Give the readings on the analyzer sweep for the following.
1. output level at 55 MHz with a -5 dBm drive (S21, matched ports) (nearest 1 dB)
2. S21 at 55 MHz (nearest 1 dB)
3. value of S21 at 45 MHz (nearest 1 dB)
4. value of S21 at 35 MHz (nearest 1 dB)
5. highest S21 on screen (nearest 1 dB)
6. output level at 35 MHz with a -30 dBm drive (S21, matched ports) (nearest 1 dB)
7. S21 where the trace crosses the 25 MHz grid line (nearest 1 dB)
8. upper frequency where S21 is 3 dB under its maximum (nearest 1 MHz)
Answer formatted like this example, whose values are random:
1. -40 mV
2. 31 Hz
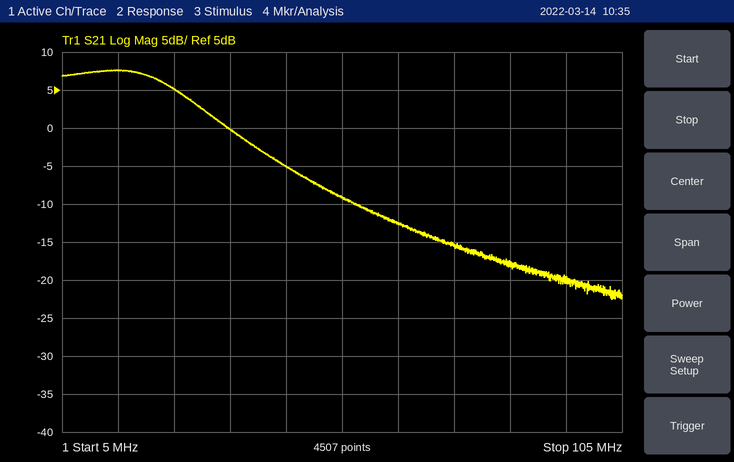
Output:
1. -14 dBm
2. -9 dB
3. -5 dB
4. 0 dB
5. 8 dB
6. -30 dBm
7. 5 dB
8. 26 MHz
